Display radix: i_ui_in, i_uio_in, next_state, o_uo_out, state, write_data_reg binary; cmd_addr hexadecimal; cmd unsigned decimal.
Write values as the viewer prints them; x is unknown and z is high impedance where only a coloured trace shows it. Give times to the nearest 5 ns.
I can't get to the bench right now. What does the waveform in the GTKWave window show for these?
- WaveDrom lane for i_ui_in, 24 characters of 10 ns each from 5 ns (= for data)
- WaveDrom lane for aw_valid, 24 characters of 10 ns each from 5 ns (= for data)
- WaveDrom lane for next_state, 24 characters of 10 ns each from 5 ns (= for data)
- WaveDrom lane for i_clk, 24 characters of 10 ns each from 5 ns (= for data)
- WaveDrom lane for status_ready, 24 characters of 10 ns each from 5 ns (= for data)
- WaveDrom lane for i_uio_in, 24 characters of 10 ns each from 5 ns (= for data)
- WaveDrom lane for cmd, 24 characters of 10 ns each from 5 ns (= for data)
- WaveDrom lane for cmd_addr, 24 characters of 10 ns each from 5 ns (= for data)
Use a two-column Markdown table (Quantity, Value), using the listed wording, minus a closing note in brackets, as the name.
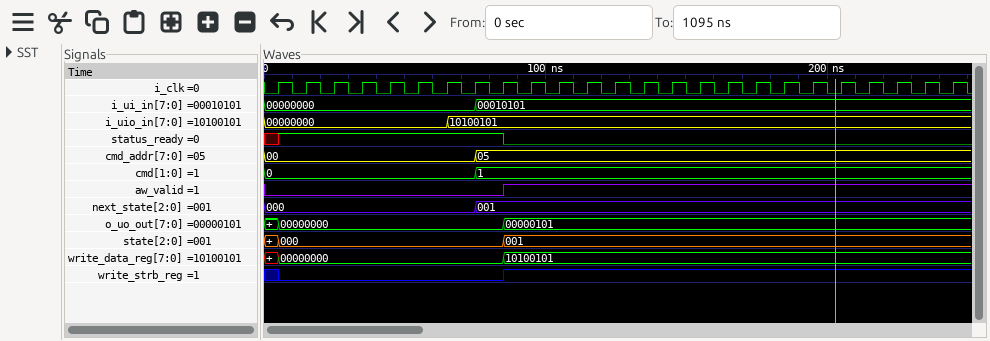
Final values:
| Quantity | Value |
|---|---|
| WaveDrom lane for i_ui_in, 24 characters of 10 ns each from 5 ns | {name: 'i_ui_in', wave: '=......=................', data: '00000000 00010101'} |
| WaveDrom lane for aw_valid, 24 characters of 10 ns each from 5 ns | {name: 'aw_valid', wave: '0.......1...............'} |
| WaveDrom lane for next_state, 24 characters of 10 ns each from 5 ns | {name: 'next_state', wave: '=......=................', data: '000 001'} |
| WaveDrom lane for i_clk, 24 characters of 10 ns each from 5 ns | {name: 'i_clk', wave: 'p.......................'} |
| WaveDrom lane for status_ready, 24 characters of 10 ns each from 5 ns | {name: 'status_ready', wave: '1.......0...............'} |
| WaveDrom lane for i_uio_in, 24 characters of 10 ns each from 5 ns | {name: 'i_uio_in', wave: '=.....=.................', data: '00000000 10100101'} |
| WaveDrom lane for cmd, 24 characters of 10 ns each from 5 ns | {name: 'cmd', wave: '=......=................', data: '0 1'} |
| WaveDrom lane for cmd_addr, 24 characters of 10 ns each from 5 ns | {name: 'cmd_addr', wave: '=......=................', data: '00 05'} |
